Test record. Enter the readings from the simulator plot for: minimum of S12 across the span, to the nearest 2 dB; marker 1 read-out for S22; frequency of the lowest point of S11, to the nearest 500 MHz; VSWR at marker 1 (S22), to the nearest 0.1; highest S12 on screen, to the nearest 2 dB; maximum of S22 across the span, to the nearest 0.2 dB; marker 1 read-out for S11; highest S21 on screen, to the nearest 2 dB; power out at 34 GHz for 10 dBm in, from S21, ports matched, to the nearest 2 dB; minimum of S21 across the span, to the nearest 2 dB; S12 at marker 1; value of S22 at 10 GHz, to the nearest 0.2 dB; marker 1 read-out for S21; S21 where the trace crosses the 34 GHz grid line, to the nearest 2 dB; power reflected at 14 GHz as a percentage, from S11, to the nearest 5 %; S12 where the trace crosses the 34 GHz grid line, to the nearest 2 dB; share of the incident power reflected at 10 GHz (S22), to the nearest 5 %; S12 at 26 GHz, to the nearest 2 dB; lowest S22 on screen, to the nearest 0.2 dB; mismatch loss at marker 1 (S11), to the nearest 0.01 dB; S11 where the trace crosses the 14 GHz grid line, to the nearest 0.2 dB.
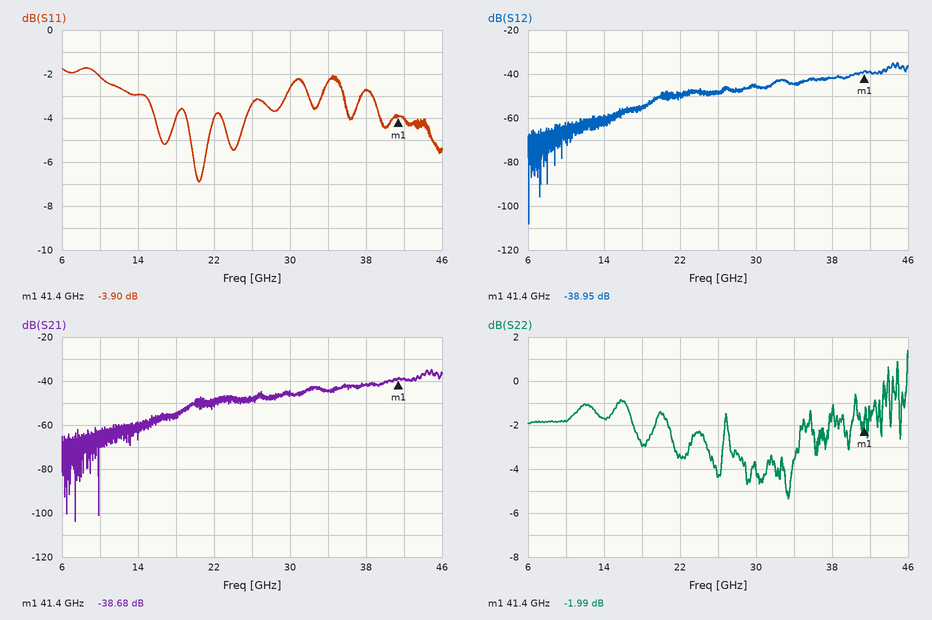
-108 dB
-1.99 dB
20.5 GHz
8.8
-34 dB
1.4 dB
-3.90 dB
-34 dB
-34 dBm
-104 dB
-38.95 dB
-1.8 dB
-38.68 dB
-44 dB
50 %
-44 dB
65 %
-48 dB
-5.4 dB
2.27 dB
-3.0 dB
